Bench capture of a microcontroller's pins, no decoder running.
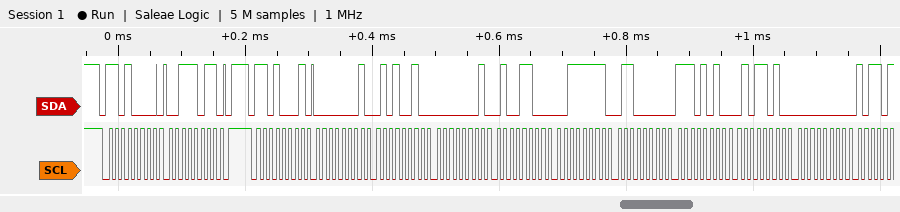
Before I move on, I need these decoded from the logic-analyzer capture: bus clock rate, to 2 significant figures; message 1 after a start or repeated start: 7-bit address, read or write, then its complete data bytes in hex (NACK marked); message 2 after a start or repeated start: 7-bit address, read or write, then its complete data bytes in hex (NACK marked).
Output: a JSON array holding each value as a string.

["100 kHz", "0x68 write: 3B", "0x68 read: 01 52 01 4C 3F 60 EA 5A 00"]
